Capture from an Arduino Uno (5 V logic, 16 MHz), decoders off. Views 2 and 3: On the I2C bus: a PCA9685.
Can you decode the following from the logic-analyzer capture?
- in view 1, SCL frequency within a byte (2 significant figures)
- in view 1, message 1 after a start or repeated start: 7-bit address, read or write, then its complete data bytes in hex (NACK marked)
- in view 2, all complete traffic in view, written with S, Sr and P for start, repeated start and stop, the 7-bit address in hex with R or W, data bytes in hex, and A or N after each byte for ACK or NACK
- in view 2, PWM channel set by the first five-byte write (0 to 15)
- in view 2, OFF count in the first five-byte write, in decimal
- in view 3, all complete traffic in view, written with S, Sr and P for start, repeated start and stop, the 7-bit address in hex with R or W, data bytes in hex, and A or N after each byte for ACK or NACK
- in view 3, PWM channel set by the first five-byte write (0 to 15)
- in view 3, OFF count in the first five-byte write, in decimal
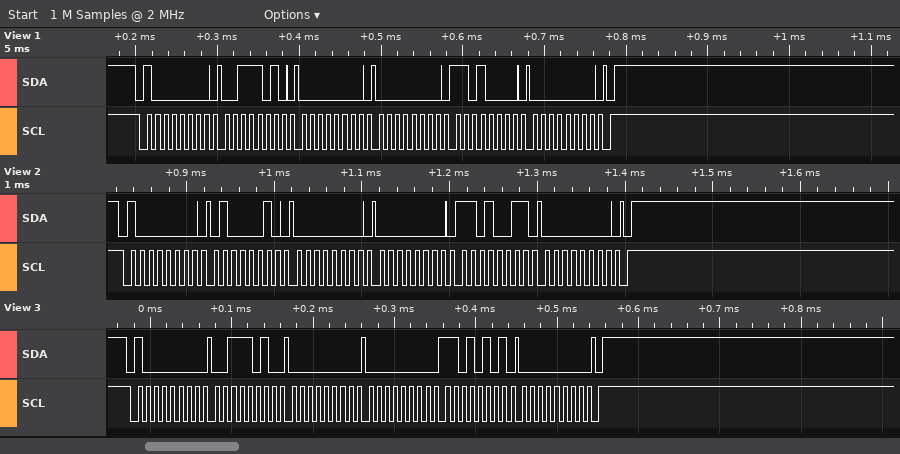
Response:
100 kHz
0x40 write: 3A 00 00 D0 00
S 40W A 42 A 00 A 00 A D3 A 00 A P
15
211
S 40W A 3A A 00 A 00 A D5 A 00 A P
13
213
